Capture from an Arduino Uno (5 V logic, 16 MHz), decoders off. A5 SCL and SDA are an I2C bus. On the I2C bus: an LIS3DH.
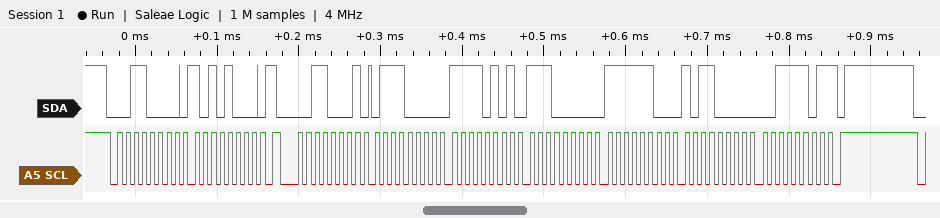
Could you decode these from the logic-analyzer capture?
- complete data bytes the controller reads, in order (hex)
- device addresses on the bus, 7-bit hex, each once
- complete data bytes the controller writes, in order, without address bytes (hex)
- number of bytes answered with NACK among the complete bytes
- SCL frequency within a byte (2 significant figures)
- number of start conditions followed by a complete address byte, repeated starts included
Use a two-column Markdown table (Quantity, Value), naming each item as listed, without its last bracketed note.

| Quantity | Value |
|---|---|
| complete data bytes the controller reads, in order | 70 F5 E0 FC B0 3D |
| device addresses on the bus, 7-bit hex, each once | 0x18 |
| complete data bytes the controller writes, in order, without address bytes | A8 |
| number of bytes answered with NACK among the complete bytes | 1 |
| SCL frequency within a byte | 100 kHz |
| number of start conditions followed by a complete address byte, repeated starts included | 2 |
